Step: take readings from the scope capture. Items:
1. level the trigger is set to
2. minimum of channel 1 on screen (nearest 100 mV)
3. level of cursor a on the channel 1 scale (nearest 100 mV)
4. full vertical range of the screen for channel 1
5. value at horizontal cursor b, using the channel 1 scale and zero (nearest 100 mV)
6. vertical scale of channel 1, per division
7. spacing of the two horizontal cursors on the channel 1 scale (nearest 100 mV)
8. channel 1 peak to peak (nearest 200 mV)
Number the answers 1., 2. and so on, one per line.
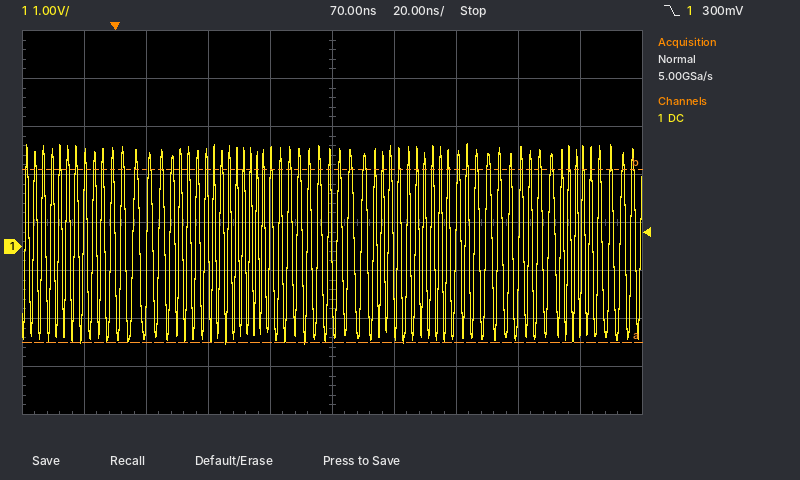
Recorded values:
1. 300 mV
2. -2.0 V
3. -2.0 V
4. 8 V
5. 1.6 V
6. 1 V
7. 3.6 V
8. 4.2 V
